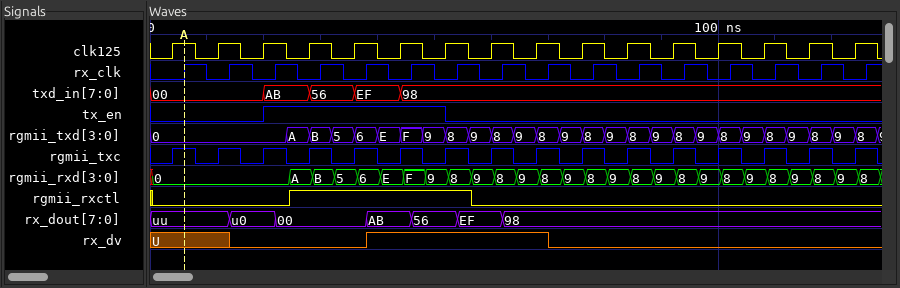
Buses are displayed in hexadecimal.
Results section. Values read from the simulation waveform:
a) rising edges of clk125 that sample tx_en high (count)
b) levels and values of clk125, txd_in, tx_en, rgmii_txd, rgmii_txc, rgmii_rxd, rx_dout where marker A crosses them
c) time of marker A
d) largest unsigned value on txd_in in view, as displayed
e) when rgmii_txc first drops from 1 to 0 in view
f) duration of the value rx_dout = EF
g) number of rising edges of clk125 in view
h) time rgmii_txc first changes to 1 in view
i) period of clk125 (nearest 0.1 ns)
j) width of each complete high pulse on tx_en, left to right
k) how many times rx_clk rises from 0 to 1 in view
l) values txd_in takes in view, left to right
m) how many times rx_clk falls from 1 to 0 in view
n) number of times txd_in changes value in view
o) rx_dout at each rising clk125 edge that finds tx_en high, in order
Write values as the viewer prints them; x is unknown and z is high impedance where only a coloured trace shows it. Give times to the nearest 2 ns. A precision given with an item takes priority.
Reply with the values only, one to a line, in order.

4
clk125=1, txd_in=00, tx_en=0, rgmii_txd=0, rgmii_txc=1, rgmii_rxd=0, rx_dout=uu
6 ns
EF
8 ns
8 ns
16
4 ns
8 ns
32 ns
16
00, AB, 56, EF, 98
15
4
00, 00, AB, 56
